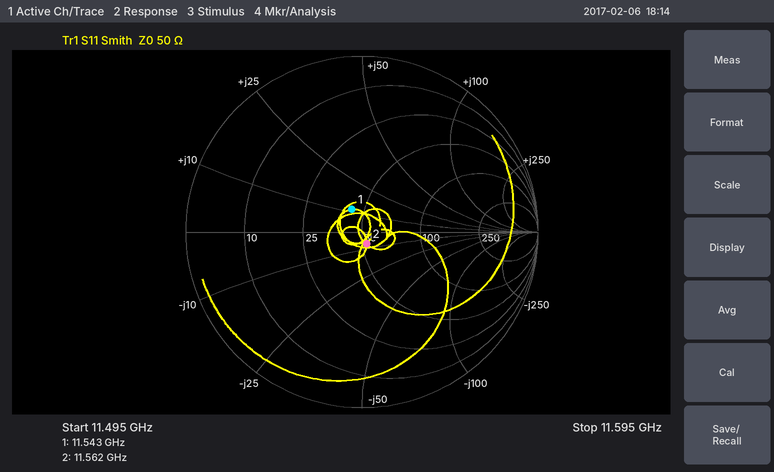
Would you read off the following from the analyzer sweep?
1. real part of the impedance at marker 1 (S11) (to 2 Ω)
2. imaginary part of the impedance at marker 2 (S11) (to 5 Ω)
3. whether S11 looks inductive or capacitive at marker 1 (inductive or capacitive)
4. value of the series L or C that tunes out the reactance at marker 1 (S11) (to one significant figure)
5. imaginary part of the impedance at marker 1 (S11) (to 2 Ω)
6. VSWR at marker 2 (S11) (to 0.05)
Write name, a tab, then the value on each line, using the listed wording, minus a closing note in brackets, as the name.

real part of the impedance at marker 1 (S11)	44 Ω
imaginary part of the impedance at marker 2 (S11)	-5 Ω
whether S11 looks inductive or capacitive at marker 1	inductive
value of the series L or C that tunes out the reactance at marker 1 (S11)	1 pF
imaginary part of the impedance at marker 1 (S11)	+12 Ω
VSWR at marker 2 (S11)	1.15
